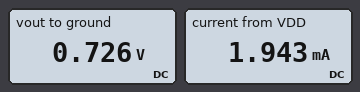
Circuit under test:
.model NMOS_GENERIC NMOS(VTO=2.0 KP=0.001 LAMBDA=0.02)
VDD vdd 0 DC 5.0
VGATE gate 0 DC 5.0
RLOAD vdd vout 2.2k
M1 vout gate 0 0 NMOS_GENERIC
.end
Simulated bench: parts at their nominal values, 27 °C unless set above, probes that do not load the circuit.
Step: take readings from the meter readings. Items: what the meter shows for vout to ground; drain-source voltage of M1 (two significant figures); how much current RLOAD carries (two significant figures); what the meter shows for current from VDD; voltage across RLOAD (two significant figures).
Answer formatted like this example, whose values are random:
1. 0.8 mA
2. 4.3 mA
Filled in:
1. 0.726 V
2. 730 mV
3. 1.9 mA
4. 1.943 mA
5. 4.3 V
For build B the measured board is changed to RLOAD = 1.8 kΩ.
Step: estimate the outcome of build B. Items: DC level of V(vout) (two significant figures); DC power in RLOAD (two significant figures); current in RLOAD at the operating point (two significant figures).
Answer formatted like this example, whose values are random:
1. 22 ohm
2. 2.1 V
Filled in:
1. 880 mV
2. 9.4 mW
3. 2.3 mA
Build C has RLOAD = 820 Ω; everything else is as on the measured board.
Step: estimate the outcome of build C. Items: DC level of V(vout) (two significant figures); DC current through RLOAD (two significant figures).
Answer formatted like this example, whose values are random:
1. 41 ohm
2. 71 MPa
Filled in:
1. 1.8 V
2. 3.9 mA
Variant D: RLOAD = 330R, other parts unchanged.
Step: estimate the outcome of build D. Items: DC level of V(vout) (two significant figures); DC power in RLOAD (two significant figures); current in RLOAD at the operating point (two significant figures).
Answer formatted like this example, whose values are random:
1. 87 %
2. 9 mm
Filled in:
1. 3.4 V
2. 7.6 mW
3. 4.8 mA
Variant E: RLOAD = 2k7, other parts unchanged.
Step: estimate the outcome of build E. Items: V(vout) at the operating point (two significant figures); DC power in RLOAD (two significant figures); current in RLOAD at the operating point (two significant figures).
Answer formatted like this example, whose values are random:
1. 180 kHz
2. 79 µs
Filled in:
1. 600 mV
2. 7.2 mW
3. 1.6 mA
